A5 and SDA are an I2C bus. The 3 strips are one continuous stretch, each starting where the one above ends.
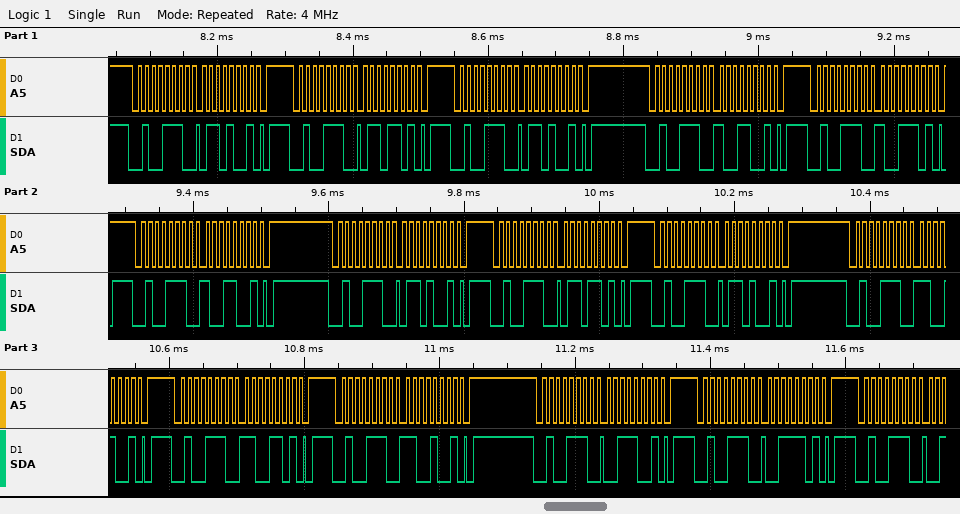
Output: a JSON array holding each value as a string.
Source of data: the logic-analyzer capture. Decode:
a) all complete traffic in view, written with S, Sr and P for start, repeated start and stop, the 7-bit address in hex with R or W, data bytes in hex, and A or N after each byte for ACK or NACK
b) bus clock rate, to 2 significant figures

["S 27W A 69 A P S 27W A 6D A P S 27W A 69 A P S 27W A 99 A P S 27W A 9D A P S 27W A 99 A P S 27W A 69 A P S 27W A 6D A P S 27W A 69 A P S 27W A C9 A P S 27W A CD A P S 27W A C9 A P S 27W A 39 A P S 27W A 3D A P S 27W A", "100 kHz"]
